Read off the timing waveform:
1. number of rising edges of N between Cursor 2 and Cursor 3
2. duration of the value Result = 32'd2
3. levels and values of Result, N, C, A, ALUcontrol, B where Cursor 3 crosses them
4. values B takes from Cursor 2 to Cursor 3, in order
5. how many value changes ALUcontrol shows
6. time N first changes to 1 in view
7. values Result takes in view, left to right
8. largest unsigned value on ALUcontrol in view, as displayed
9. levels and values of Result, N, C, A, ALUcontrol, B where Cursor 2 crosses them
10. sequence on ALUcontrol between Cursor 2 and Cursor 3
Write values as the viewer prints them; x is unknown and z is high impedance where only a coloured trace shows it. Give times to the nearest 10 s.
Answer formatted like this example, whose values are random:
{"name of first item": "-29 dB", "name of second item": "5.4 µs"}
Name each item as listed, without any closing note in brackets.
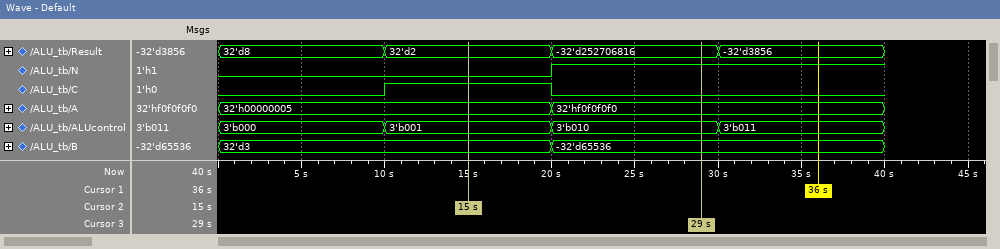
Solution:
{"number of rising edges of N between Cursor 2 and Cursor 3": "1", "duration of the value Result = 32'd2": "10 s", "levels and values of Result, N, C, A, ALUcontrol, B where Cursor 3 crosses them": "Result=-32'd252706816, N=1, C=0, A=32'hf0f0f0f0, ALUcontrol=3'b010, B=-32'd65536", "values B takes from Cursor 2 to Cursor 3, in order": "32'd3, -32'd65536", "how many value changes ALUcontrol shows": "3", "time N first changes to 1 in view": "20 s", "values Result takes in view, left to right": "32'd8, 32'd2, -32'd252706816, -32'd3856", "largest unsigned value on ALUcontrol in view, as displayed": "3'b011", "levels and values of Result, N, C, A, ALUcontrol, B where Cursor 2 crosses them": "Result=32'd2, N=0, C=1, A=32'h00000005, ALUcontrol=3'b001, B=32'd3", "sequence on ALUcontrol between Cursor 2 and Cursor 3": "3'b001, 3'b010"}
